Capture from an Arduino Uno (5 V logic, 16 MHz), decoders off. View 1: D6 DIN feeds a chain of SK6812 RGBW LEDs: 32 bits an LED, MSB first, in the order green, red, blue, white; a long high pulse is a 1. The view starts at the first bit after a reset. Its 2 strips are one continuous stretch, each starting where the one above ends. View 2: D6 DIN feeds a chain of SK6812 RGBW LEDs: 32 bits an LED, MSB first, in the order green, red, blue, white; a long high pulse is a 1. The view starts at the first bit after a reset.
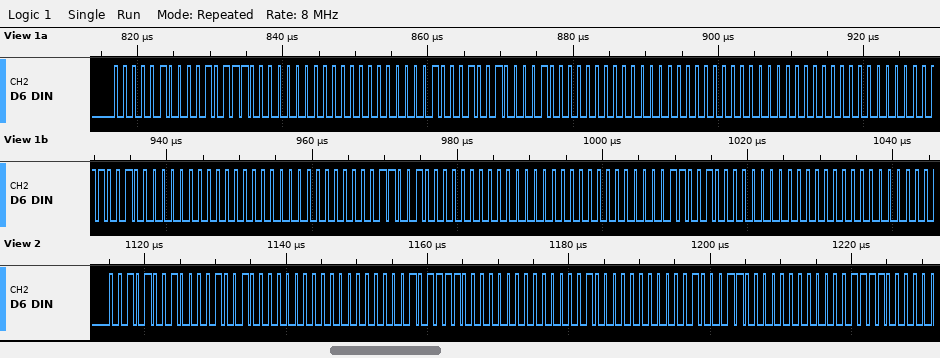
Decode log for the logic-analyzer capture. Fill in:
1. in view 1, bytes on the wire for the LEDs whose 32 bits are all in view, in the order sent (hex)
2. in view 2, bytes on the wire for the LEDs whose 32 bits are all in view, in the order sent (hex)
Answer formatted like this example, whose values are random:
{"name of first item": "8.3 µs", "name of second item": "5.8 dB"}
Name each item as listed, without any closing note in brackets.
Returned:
{"in view 1, bytes on the wire for the LEDs whose 32 bits are all in view, in the order sent": "04 2E 00 00 11 21 00 00 00 00 00 32 00 00 00 32 00 00 00 32", "in view 2, bytes on the wire for the LEDs whose 32 bits are all in view, in the order sent": "29 09 00 00 2F 00 02 00"}
